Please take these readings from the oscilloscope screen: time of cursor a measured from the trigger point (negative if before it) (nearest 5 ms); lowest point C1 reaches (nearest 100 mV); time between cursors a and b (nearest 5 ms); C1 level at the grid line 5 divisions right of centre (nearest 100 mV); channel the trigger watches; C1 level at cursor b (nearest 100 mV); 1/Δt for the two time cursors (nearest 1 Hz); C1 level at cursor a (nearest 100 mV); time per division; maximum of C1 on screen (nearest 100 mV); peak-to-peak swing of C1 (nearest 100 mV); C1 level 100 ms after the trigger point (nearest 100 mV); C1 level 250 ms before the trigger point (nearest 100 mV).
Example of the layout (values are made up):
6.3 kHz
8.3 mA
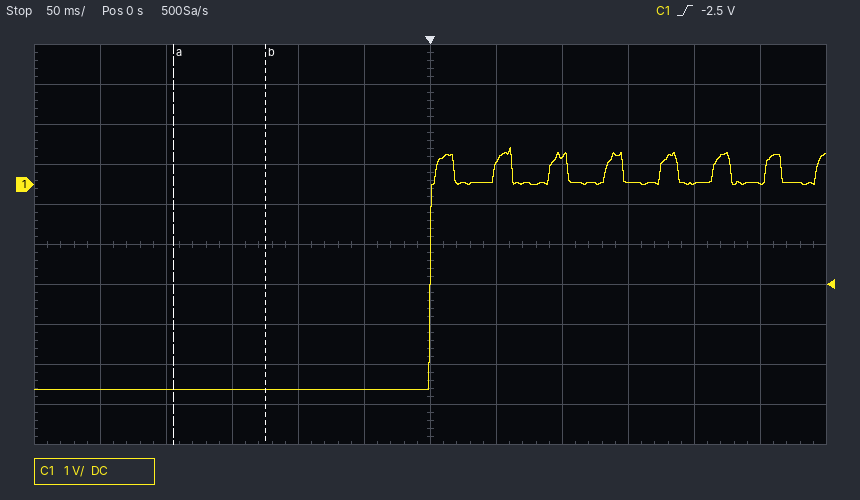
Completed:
-195 ms
-5.1 V
70 ms
0.0 V
C1
-5.1 V
14 Hz
-5.1 V
50 ms
900 mV
6.0 V
700 mV
-5.1 V
